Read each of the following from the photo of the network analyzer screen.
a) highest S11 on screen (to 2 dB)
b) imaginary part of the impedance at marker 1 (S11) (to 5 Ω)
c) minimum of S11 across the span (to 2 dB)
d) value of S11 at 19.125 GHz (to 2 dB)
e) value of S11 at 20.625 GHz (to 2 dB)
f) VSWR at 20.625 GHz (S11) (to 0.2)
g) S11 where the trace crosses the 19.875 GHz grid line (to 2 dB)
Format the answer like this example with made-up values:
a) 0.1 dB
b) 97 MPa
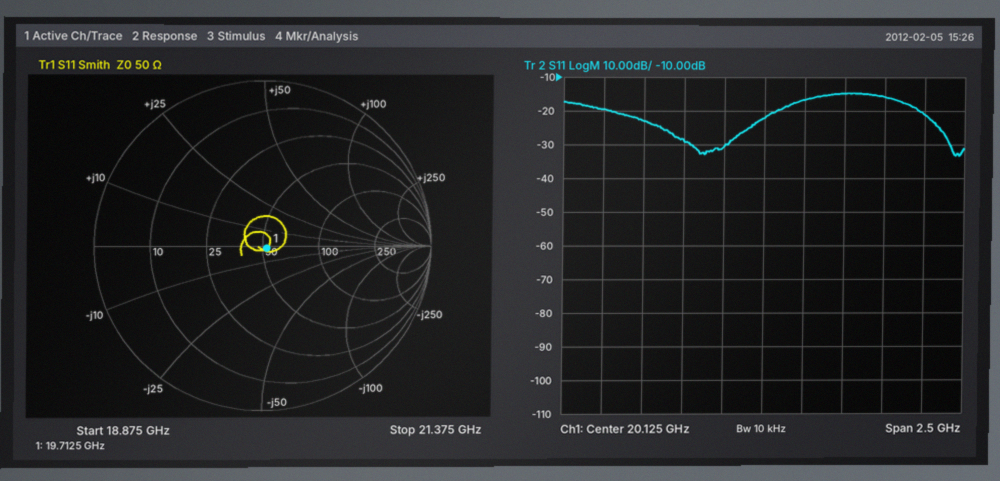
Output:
a) -14 dB
b) 0 Ω
c) -34 dB
d) -20 dB
e) -14 dB
f) 1.4
g) -30 dB
